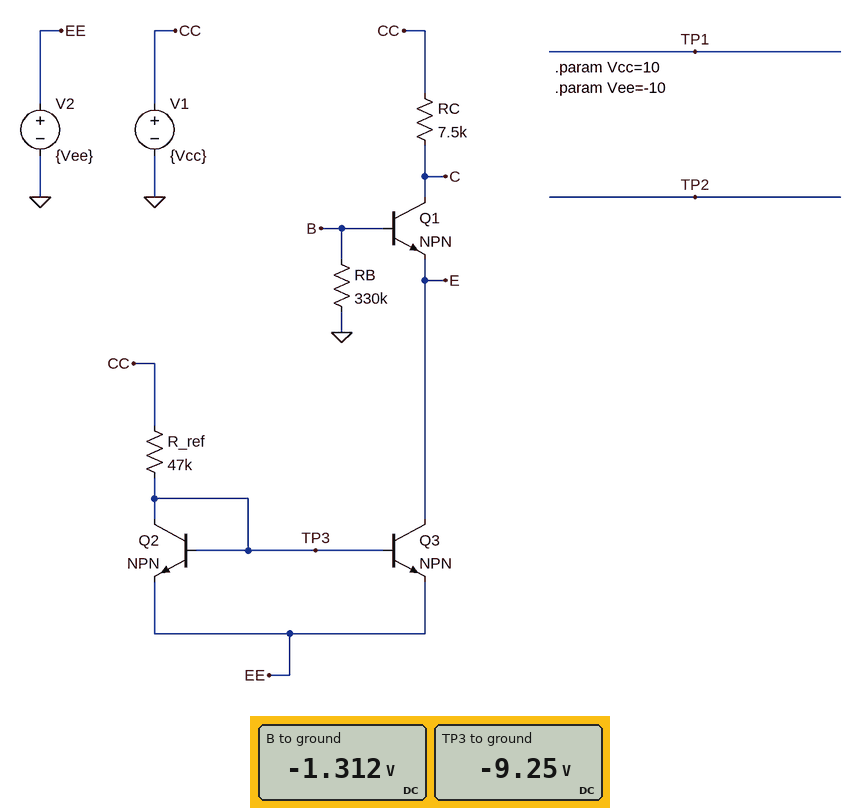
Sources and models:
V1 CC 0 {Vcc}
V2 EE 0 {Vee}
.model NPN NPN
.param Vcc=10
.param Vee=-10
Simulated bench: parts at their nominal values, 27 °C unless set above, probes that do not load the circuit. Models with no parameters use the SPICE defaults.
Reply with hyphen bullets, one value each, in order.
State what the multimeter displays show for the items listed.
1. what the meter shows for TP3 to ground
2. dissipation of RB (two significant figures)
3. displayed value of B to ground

- -9.25 V
- 5.2 µW
- -1.312 V
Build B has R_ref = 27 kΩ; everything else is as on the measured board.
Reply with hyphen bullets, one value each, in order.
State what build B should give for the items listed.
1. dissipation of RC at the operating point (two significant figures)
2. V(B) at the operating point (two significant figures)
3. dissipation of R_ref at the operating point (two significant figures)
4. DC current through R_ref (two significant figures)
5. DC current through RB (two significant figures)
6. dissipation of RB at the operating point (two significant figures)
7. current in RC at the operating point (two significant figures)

- 3.6 mW
- -2.3 V
- 14 mW
- 710 µA
- 6.9 µA
- 16 µW
- 690 µA
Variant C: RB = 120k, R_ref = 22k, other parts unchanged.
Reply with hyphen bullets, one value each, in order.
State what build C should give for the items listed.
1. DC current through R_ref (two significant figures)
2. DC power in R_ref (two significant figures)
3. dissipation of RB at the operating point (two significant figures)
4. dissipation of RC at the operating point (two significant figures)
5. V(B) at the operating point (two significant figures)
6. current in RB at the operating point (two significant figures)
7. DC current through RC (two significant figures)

- 870 µA
- 17 mW
- 8.6 µW
- 5.4 mW
- -1.0 V
- 8.5 µA
- 850 µA
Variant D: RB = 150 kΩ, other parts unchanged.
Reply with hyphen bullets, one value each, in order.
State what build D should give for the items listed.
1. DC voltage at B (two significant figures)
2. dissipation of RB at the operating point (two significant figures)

- -600 mV
- 2.4 µW
